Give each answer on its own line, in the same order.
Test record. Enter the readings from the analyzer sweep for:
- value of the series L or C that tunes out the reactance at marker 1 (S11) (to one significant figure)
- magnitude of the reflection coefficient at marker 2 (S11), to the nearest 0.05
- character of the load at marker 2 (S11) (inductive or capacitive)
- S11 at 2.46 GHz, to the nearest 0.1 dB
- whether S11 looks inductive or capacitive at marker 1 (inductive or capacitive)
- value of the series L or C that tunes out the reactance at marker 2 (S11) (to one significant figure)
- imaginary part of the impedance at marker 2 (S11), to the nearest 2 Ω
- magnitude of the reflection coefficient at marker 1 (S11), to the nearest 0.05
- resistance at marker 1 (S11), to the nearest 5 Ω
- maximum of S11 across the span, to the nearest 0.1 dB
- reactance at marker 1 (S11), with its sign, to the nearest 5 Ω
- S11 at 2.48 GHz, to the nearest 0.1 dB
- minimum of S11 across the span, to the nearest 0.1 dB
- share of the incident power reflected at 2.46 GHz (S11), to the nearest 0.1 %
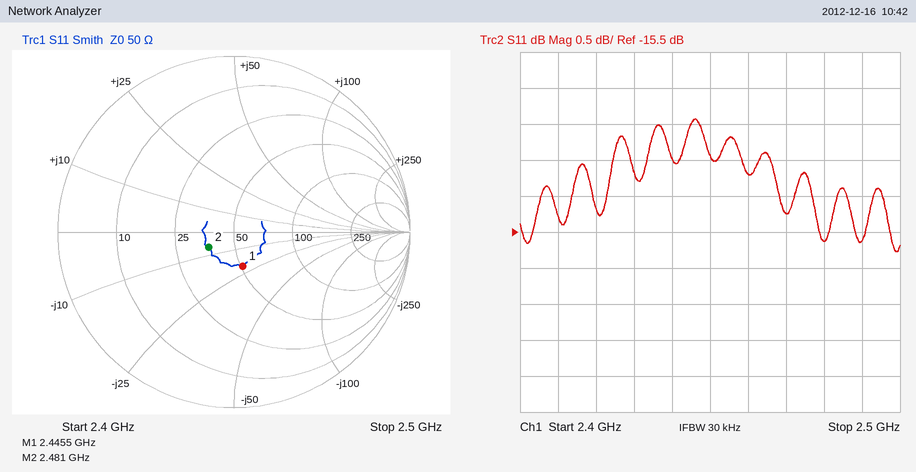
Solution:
1 nH
0.15
capacitive
-14.7 dB
capacitive
400 pH
-6 Ω
0.20
50 Ω
-13.9 dB
-20 Ω
-15.6 dB
-15.8 dB
3.4 %
